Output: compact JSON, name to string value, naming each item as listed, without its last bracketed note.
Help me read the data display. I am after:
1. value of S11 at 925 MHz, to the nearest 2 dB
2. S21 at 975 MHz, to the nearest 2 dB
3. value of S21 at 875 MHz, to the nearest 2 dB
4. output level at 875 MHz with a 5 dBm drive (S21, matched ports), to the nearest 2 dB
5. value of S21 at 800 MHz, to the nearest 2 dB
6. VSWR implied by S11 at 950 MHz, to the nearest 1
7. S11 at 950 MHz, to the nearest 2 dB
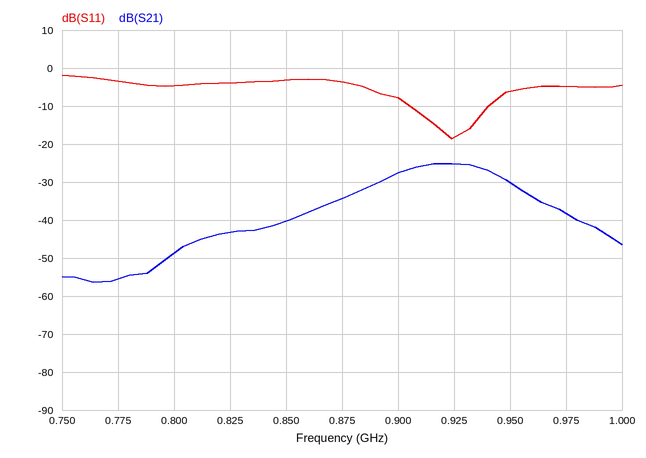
{"value of S11 at 925 MHz, to the nearest 2 dB": "-18 dB", "S21 at 975 MHz, to the nearest 2 dB": "-38 dB", "value of S21 at 875 MHz, to the nearest 2 dB": "-34 dB", "output level at 875 MHz with a 5 dBm drive (S21, matched ports), to the nearest 2 dB": "-30 dBm", "value of S21 at 800 MHz, to the nearest 2 dB": "-48 dB", "VSWR implied by S11 at 950 MHz, to the nearest 1": "3", "S11 at 950 MHz, to the nearest 2 dB": "-6 dB"}
